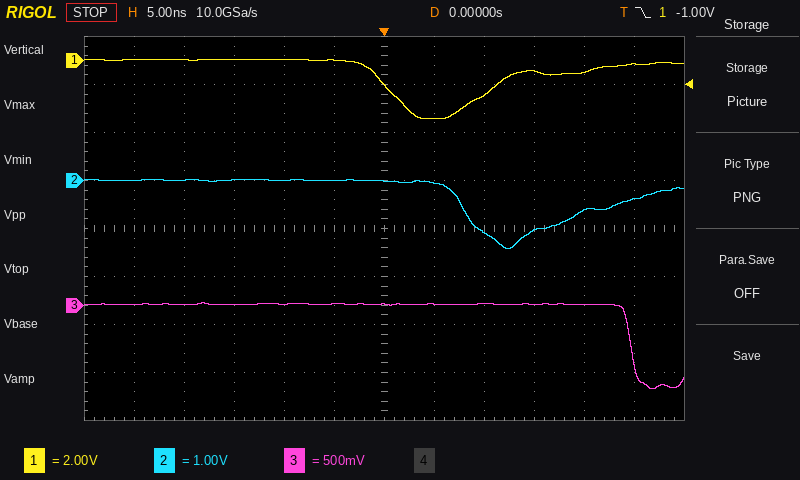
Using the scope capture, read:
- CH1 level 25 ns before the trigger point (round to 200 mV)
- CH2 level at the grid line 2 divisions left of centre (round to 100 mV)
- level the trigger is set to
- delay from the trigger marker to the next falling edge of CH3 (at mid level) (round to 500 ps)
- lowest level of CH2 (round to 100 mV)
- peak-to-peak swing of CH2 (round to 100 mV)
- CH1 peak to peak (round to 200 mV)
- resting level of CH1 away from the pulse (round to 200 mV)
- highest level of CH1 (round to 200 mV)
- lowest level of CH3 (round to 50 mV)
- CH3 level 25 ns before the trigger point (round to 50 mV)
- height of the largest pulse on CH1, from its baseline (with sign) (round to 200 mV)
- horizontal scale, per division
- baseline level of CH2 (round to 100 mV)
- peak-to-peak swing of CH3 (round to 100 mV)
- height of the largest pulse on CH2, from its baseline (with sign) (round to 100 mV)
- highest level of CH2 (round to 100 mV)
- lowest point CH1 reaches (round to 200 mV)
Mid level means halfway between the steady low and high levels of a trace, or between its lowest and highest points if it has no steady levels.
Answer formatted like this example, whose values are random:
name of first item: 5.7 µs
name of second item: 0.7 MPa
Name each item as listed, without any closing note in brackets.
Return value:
CH1 level 25 ns before the trigger point: 0.0 V
CH2 level at the grid line 2 divisions left of centre: 0.0 V
level the trigger is set to: -1.00 V
delay from the trigger marker to the next falling edge of CH3 (at mid level): 24.5 ns
lowest level of CH2: -1.4 V
peak-to-peak swing of CH2: 1.4 V
CH1 peak to peak: 2.4 V
resting level of CH1 away from the pulse: 0.0 V
highest level of CH1: 0.0 V
lowest level of CH3: -850 mV
CH3 level 25 ns before the trigger point: 0 mV
height of the largest pulse on CH1, from its baseline (with sign): -2.4 V
horizontal scale, per division: 5 ns
baseline level of CH2: 0.0 V
peak-to-peak swing of CH3: 900 mV
height of the largest pulse on CH2, from its baseline (with sign): -1.4 V
highest level of CH2: 0.0 V
lowest point CH1 reaches: -2.4 V
